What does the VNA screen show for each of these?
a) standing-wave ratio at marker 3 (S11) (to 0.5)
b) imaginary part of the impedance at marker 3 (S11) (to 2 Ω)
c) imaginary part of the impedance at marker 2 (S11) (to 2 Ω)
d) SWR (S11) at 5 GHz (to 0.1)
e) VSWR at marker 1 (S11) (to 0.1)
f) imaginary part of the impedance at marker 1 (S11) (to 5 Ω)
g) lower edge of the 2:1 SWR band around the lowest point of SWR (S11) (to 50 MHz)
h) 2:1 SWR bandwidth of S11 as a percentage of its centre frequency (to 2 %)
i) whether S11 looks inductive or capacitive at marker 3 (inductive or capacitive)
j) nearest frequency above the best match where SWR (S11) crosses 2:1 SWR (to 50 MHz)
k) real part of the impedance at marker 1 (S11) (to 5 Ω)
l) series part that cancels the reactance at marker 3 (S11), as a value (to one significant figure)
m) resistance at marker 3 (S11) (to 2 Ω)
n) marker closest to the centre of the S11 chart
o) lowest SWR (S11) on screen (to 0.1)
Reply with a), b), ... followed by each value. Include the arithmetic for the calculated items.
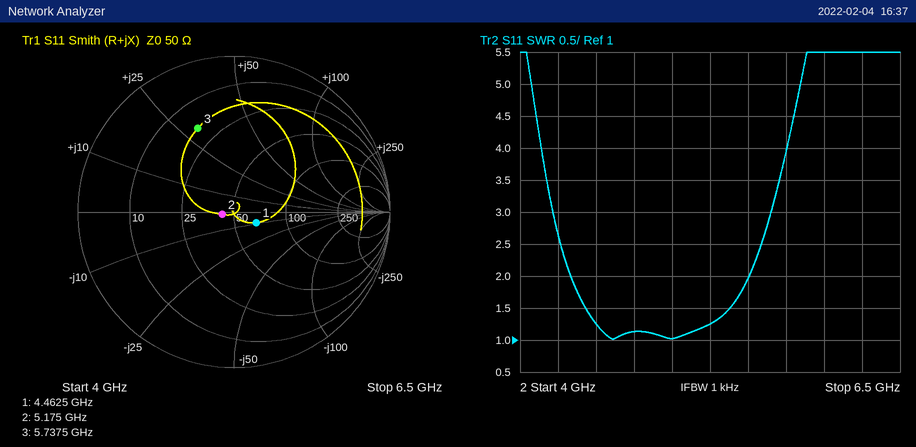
a) 4.0
b) +30 Ω
c) -2 Ω
d) 1.0
e) 1.4
f) -10 Ω
g) 4.35 GHz
h) 1.15 GHz / 4.925 GHz ≈ 23.4 %, so 24 % to the nearest 2 %
i) inductive
j) 5.50 GHz
k) 65 Ω
l) C = 1/(2π × 5.7375 GHz × 30 Ω) ≈ 925 fF, so 900 fF to one significant figure
m) 18 Ω
n) marker 2
o) 1.0
